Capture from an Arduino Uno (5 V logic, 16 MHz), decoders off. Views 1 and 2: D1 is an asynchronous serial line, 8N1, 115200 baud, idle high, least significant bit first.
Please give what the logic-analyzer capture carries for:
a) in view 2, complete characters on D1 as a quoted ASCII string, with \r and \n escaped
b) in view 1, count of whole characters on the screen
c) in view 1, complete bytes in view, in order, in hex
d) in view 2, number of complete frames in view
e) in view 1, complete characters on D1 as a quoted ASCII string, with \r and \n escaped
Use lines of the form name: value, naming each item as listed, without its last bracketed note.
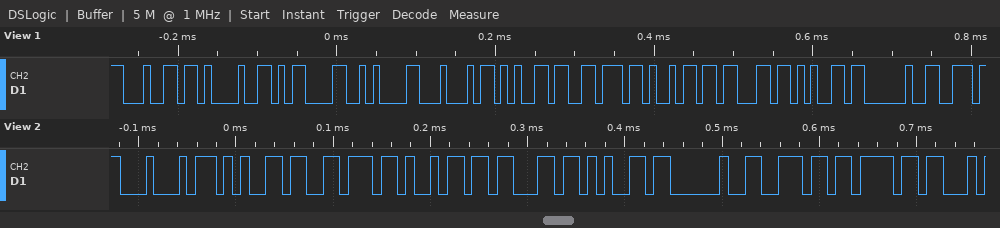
in view 2, complete characters on D1 as a quoted ASCII string, with \r and \n escaped: "Device no"
in view 1, count of whole characters on the screen: 11
in view 1, complete bytes in view, in order, in hex: 0x64 0x21 0x0D 0x0A 0x44 0x65 0x76 0x69 0x63 0x65 0x20
in view 2, number of complete frames in view: 9
in view 1, complete characters on D1 as a quoted ASCII string, with \r and \n escaped: "d!\r\nDevice "
